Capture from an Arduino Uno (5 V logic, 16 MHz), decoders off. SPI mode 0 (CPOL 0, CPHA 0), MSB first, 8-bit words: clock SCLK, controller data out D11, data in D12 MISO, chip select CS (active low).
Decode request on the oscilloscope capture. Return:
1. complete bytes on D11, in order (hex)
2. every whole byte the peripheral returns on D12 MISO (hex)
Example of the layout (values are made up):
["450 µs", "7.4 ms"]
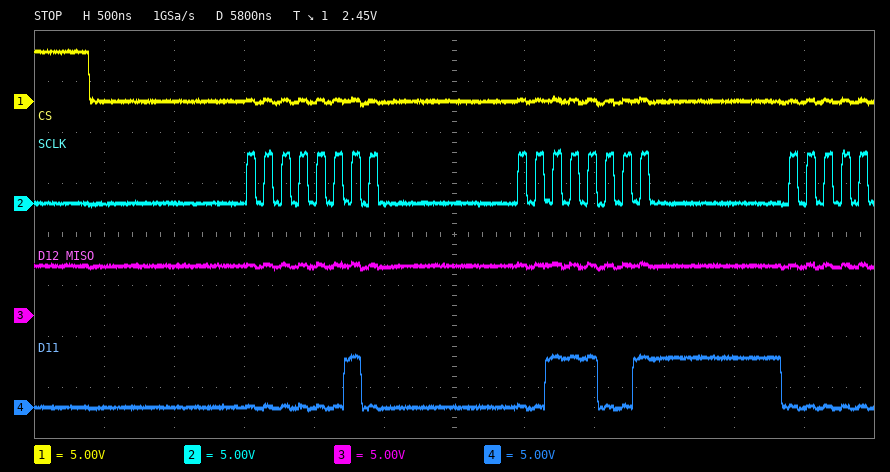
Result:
["0x02 0x39", "0xFF 0xFF"]
